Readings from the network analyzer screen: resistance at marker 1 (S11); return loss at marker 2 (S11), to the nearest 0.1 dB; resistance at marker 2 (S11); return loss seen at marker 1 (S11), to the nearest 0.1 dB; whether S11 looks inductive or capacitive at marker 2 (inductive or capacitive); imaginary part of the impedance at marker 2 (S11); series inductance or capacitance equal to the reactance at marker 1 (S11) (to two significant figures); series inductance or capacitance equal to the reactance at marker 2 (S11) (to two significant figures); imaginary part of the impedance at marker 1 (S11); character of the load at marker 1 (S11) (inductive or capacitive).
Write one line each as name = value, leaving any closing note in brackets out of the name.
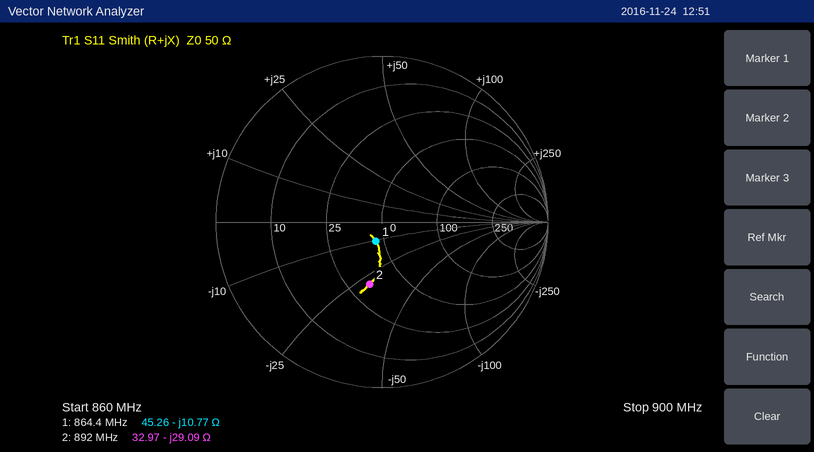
resistance at marker 1 = 45.26 Ω
return loss at marker 2 (S11), to the nearest 0.1 dB = 8.3 dB
resistance at marker 2 = 32.97 Ω
return loss seen at marker 1 (S11), to the nearest 0.1 dB = 18.2 dB
whether S11 looks inductive or capacitive at marker 2 = capacitive
imaginary part of the impedance at marker 2 = -29.09 Ω
series inductance or capacitance equal to the reactance at marker 1 (S11) = 17 pF
series inductance or capacitance equal to the reactance at marker 2 (S11) = 6.1 pF
imaginary part of the impedance at marker 1 = -10.77 Ω
character of the load at marker 1 (S11) = capacitive
